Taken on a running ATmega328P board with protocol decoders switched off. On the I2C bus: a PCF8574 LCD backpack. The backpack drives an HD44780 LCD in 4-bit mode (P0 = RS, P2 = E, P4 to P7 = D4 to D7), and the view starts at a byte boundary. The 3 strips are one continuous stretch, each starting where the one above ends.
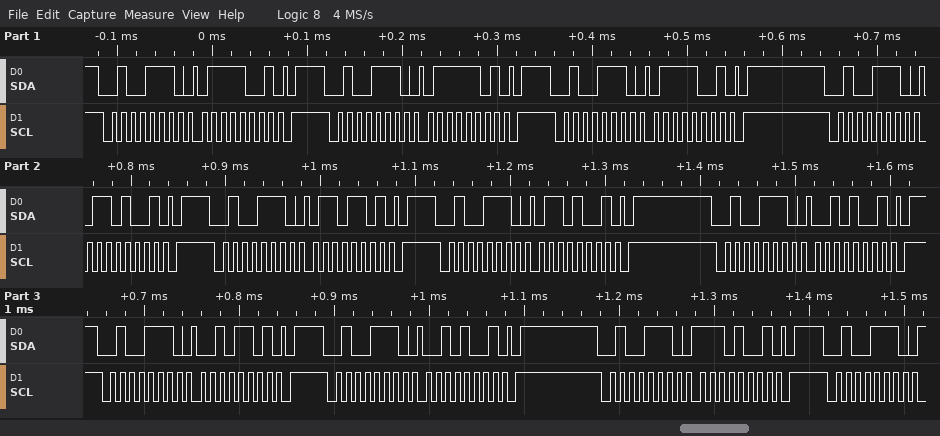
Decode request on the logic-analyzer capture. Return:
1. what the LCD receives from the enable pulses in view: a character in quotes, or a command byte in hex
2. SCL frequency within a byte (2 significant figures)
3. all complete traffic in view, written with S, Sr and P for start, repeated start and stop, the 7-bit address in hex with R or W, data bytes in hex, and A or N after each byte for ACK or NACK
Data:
'v'
100 kHz
S 27W A 79 A P S 27W A 7D A P S 27W A 79 A P S 27W A 69 A P S 27W A 6D A P S 27W A 69 A P S 27W A 29 A P S 27W A 2D A P S 27W A 29 A P S 27W A E9 A P S 27W A
